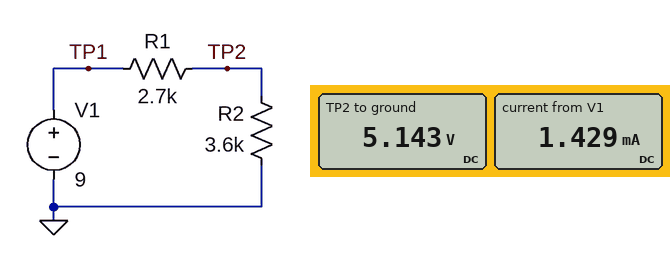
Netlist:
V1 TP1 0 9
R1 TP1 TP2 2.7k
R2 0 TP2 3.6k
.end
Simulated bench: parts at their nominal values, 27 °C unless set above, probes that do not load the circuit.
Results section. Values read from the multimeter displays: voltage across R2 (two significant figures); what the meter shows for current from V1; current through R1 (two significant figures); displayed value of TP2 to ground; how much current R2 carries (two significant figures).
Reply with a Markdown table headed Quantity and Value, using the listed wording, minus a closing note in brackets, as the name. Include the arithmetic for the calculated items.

| Quantity | Value |
|---|---|
| voltage across R2 | 5.143 V = 5.1 V |
| what the meter shows for current from V1 | 1.429 mA |
| current through R1 | (9 V - 5.143 V) / 2.7 kΩ = 1.4 mA |
| displayed value of TP2 to ground | 5.143 V |
| how much current R2 carries | (5.143 V) / 3.6 kΩ = 1.4 mA |
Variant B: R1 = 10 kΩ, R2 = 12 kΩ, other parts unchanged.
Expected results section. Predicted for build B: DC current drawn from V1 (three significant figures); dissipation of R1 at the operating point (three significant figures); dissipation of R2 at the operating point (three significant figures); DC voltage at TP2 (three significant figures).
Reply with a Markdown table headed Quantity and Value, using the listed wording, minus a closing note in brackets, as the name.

| Quantity | Value |
|---|---|
| DC current drawn from V1 | 409 µA |
| dissipation of R1 at the operating point | 1.67 mW |
| dissipation of R2 at the operating point | 2.01 mW |
| DC voltage at TP2 | 4.91 V |
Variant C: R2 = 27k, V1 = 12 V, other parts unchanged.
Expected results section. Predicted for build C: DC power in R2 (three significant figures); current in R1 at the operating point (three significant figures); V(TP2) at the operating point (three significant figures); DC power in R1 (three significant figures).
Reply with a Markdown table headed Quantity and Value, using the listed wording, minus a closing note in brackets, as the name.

| Quantity | Value |
|---|---|
| DC power in R2 | 4.41 mW |
| current in R1 at the operating point | 404 µA |
| V(TP2) at the operating point | 10.9 V |
| DC power in R1 | 441 µW |
